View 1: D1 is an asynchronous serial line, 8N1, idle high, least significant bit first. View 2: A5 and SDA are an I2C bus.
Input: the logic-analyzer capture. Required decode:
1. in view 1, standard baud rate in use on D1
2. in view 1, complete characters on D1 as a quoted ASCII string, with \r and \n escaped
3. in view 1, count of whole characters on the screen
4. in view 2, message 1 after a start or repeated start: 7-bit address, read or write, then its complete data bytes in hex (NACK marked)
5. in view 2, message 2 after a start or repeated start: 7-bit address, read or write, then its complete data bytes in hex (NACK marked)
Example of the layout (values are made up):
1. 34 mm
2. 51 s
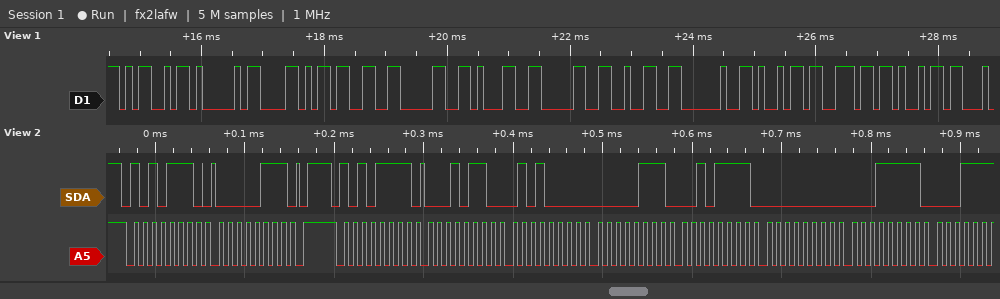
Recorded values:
1. 9600 baud
2. "MAX30102 ini"
3. 12
4. 0x57 write: 07
5. 0x57 read: 16 50 07 2F 00 1F
